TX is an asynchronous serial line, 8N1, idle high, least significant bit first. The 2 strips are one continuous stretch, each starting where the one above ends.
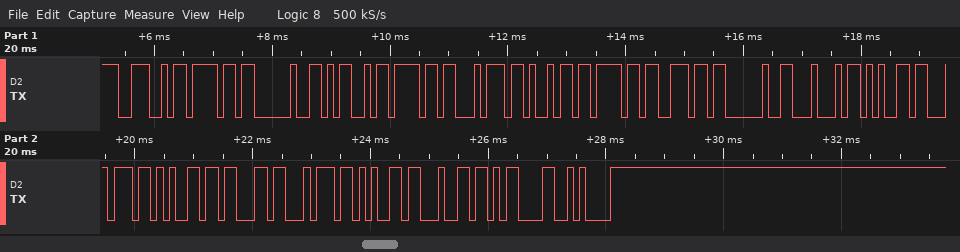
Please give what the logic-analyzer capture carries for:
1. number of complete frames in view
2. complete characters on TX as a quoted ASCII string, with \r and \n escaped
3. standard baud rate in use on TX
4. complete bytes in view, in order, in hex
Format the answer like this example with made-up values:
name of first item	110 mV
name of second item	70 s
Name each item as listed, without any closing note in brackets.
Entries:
number of complete frames in view	20
complete characters on TX as a quoted ASCII string, with \r and \n escaped	"No Motion Detected\r\n"
standard baud rate in use on TX	9600 baud
complete bytes in view, in order, in hex	4E 6F 20 4D 6F 74 69 6F 6E 20 44 65 74 65 63 74 65 64 0D 0A
